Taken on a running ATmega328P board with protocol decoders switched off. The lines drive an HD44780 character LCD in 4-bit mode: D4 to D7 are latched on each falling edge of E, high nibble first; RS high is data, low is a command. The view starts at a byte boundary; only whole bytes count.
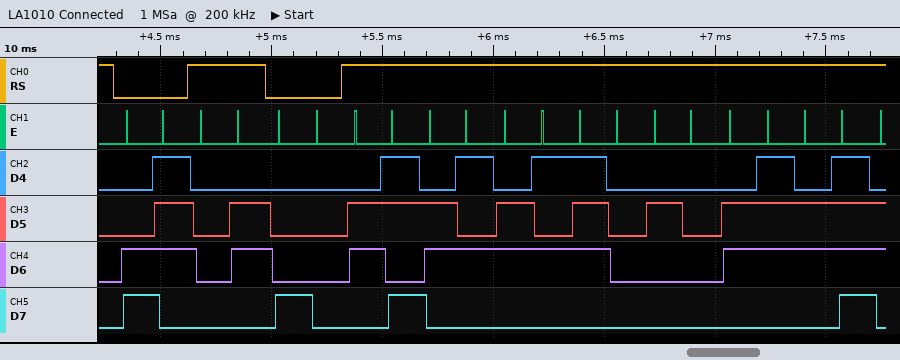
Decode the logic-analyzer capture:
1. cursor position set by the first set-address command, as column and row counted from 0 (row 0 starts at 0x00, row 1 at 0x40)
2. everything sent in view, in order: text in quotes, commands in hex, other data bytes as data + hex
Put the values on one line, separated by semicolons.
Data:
column 7, row 1; 0xC7 data 06 0x80 "keep go"
